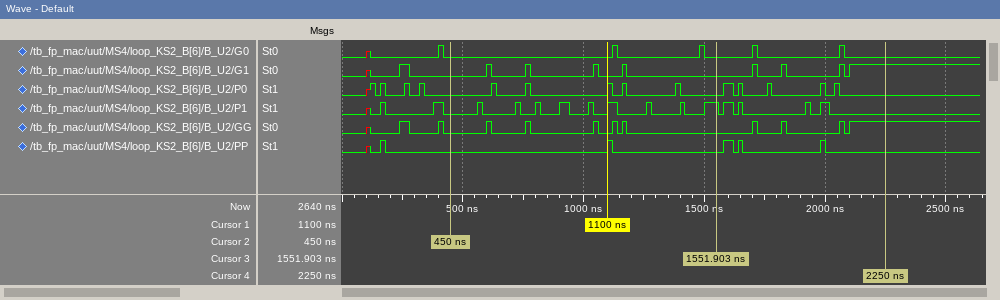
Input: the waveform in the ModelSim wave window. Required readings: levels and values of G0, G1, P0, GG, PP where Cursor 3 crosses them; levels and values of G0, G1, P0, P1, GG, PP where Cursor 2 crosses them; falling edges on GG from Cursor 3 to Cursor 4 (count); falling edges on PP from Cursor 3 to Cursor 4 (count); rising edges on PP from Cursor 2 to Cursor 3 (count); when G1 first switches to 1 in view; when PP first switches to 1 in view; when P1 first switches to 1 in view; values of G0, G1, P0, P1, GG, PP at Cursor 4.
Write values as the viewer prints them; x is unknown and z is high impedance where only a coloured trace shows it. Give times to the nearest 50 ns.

G0=0, G1=0, P0=0, GG=0, PP=0
G0=0, G1=0, P0=0, P1=0, GG=0, PP=0
3
3
1
250 ns
150 ns
150 ns
G0=0, G1=1, P0=0, P1=0, GG=1, PP=0
